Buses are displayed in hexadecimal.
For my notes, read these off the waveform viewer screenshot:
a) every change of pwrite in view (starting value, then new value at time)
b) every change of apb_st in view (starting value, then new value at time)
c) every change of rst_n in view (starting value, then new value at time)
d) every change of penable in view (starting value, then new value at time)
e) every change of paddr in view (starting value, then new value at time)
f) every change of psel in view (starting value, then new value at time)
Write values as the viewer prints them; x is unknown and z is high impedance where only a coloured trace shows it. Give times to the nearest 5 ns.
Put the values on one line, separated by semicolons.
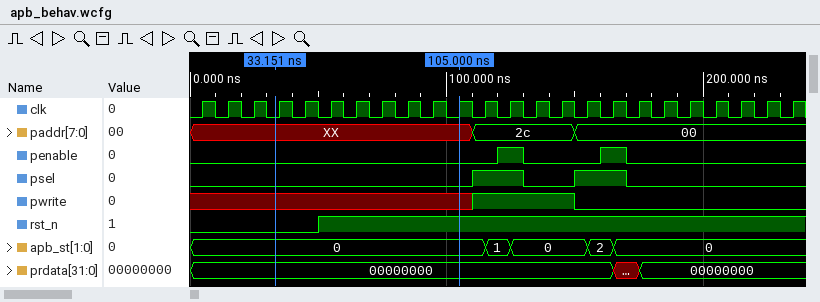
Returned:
x, 1 at 110 ns, 0 at 150 ns; 0, 1 at 115 ns, 0 at 125 ns, 2 at 155 ns, 0 at 165 ns; 0, 1 at 50 ns; 0, 1 at 120 ns, 0 at 130 ns, 1 at 160 ns, 0 at 170 ns; XX, 2c at 110 ns, 00 at 150 ns; 0, 1 at 110 ns, 0 at 130 ns, 1 at 150 ns, 0 at 170 ns
